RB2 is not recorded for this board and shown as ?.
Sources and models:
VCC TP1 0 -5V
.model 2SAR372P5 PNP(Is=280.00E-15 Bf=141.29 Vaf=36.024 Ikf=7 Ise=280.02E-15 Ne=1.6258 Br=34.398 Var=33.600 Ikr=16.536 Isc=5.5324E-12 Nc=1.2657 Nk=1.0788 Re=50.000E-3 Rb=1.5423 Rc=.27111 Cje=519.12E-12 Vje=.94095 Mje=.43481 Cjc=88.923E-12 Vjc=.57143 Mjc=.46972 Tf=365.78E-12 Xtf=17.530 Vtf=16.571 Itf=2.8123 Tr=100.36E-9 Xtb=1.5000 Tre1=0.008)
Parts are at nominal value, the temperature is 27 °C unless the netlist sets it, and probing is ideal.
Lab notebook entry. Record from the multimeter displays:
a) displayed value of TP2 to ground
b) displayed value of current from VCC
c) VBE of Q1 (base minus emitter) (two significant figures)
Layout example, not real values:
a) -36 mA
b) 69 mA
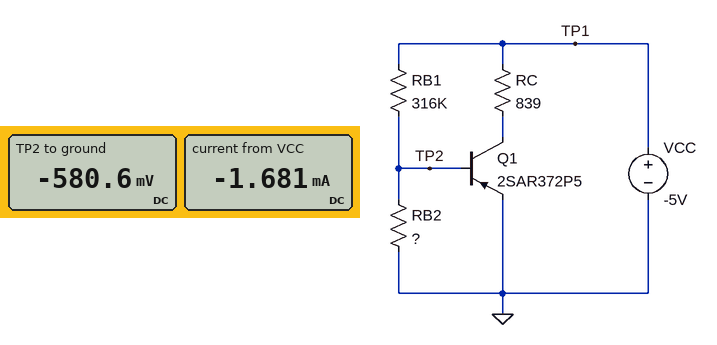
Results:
a) -580.6 mV
b) -1.681 mA
c) -580 mV
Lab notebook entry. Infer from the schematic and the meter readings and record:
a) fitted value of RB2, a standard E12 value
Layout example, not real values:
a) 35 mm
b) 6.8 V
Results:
a) 220 kΩ
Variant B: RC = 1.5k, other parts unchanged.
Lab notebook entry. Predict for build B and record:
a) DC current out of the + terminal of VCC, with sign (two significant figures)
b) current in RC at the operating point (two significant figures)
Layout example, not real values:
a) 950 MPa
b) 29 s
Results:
a) -1.6 mA
b) 1.6 mA
